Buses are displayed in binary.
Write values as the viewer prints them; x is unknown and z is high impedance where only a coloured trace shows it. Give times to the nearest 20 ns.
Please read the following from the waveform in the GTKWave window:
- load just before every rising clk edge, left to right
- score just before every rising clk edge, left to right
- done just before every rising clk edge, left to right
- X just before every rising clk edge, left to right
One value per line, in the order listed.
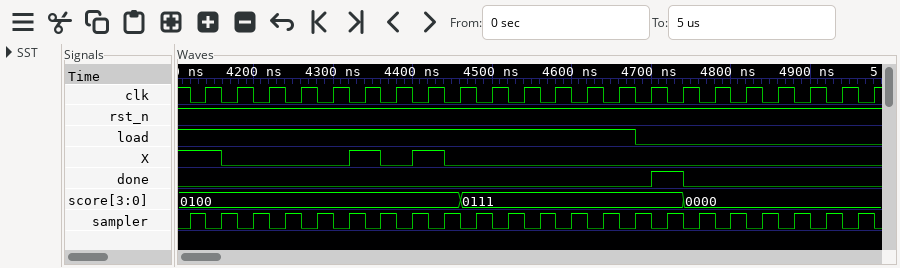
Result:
1 1 1 1 1 1 1 1 1 1 1 1 1 1 0 0 0 0 0 0 0 0
0100, 0100, 0100, 0100, 0100, 0100, 0100, 0100, 0100, 0111, 0111, 0111, 0111, 0111, 0111, 0111, 0000, 0000, 0000, 0000, 0000, 0000
0 0 0 0 0 0 0 0 0 0 0 0 0 0 0 1 0 0 0 0 0 0
1 0 0 0 0 1 0 1 0 0 0 0 0 0 0 0 0 0 0 0 0 0
